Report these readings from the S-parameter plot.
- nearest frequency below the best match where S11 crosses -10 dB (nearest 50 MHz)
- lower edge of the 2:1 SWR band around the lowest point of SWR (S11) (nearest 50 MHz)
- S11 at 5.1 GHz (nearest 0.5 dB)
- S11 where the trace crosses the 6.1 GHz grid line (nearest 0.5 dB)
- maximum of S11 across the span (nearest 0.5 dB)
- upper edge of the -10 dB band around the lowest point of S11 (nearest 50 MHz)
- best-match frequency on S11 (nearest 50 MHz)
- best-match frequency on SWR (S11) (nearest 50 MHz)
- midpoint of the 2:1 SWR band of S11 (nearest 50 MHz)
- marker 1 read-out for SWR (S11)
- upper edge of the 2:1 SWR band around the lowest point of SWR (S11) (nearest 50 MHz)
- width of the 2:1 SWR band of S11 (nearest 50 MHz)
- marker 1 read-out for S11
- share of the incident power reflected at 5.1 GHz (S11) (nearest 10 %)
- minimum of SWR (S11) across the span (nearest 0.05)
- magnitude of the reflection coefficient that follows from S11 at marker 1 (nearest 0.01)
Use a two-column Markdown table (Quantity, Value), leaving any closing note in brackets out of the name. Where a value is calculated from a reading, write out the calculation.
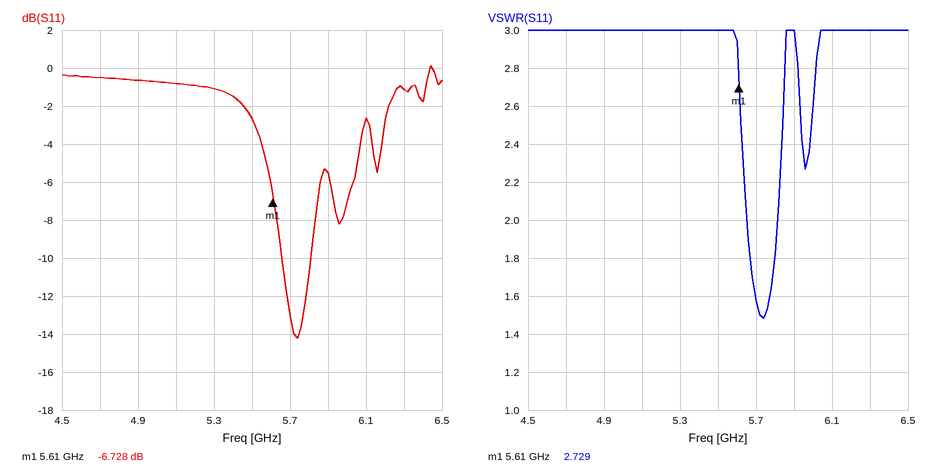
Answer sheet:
| Quantity | Value |
|---|---|
| nearest frequency below the best match where S11 crosses -10 dB | 5.65 GHz |
| lower edge of the 2:1 SWR band around the lowest point of SWR (S11) | 5.65 GHz |
| S11 at 5.1 GHz | -1.0 dB |
| S11 where the trace crosses the 6.1 GHz grid line | -2.5 dB |
| maximum of S11 across the span | 0.0 dB |
| upper edge of the -10 dB band around the lowest point of S11 | 5.80 GHz |
| best-match frequency on S11 | 5.75 GHz |
| best-match frequency on SWR (S11) | 5.75 GHz |
| midpoint of the 2:1 SWR band of S11 | 5.75 GHz |
| marker 1 read-out for SWR | 2.729 |
| upper edge of the 2:1 SWR band around the lowest point of SWR (S11) | 5.80 GHz |
| width of the 2:1 SWR band of S11 | 5.80 GHz − 5.65 GHz = 150 MHz |
| marker 1 read-out for S11 | -6.728 dB |
| share of the incident power reflected at 5.1 GHz (S11) | 10^(-1/10) ≈ 79.4 %, so 80 % to the nearest 10 % |
| minimum of SWR (S11) across the span | 1.50 |
| magnitude of the reflection coefficient that follows from S11 at marker 1 | 10^(-6.728/20) ≈ 0.46 |
